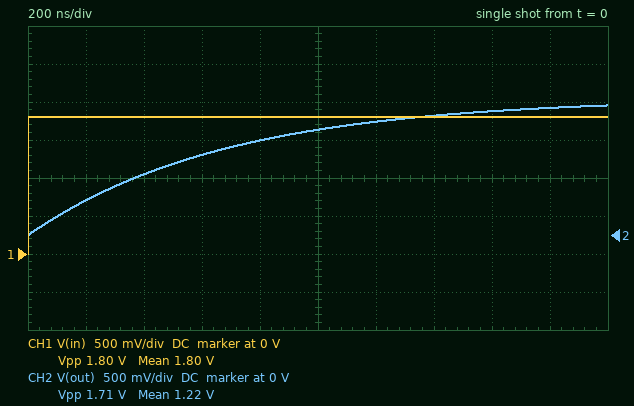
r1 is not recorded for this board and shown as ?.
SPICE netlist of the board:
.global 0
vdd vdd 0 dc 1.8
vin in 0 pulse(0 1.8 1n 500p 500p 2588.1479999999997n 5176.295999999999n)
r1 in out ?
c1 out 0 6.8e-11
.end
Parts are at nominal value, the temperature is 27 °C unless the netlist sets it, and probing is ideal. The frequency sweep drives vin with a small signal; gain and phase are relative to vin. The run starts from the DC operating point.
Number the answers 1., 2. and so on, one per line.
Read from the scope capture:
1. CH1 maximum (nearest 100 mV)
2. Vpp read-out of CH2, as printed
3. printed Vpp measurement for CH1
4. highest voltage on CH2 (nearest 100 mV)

1. 1.8 V
2. 1.71 V
3. 1.80 V
4. 1.7 V
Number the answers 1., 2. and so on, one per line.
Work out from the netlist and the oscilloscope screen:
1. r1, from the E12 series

1. 10 kΩ
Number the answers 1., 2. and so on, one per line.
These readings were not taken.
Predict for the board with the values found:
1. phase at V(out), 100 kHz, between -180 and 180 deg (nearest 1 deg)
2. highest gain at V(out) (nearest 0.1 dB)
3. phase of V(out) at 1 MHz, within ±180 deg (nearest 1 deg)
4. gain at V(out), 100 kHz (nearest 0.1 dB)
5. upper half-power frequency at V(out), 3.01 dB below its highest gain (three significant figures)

1. -23 deg
2. 0 dB
3. -77 deg
4. -0.7 dB
5. 234 kHz
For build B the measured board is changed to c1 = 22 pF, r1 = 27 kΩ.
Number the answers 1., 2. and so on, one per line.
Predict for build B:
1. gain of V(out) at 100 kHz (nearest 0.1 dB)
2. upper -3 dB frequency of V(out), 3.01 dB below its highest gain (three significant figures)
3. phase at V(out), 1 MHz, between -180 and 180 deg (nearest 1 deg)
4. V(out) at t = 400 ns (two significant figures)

1. -0.6 dB
2. 268 kHz
3. -75 deg
4. 880 mV
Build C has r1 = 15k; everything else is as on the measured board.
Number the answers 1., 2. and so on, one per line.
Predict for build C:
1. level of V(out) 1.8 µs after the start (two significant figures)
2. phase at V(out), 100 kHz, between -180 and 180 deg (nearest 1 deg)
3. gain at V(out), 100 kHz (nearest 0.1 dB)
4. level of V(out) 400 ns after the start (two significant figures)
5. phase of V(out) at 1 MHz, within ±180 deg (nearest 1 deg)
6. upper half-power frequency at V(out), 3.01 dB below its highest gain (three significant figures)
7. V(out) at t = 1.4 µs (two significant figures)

1. 1.5 V
2. -33 deg
3. -1.5 dB
4. 580 mV
5. -81 deg
6. 156 kHz
7. 1.3 V
